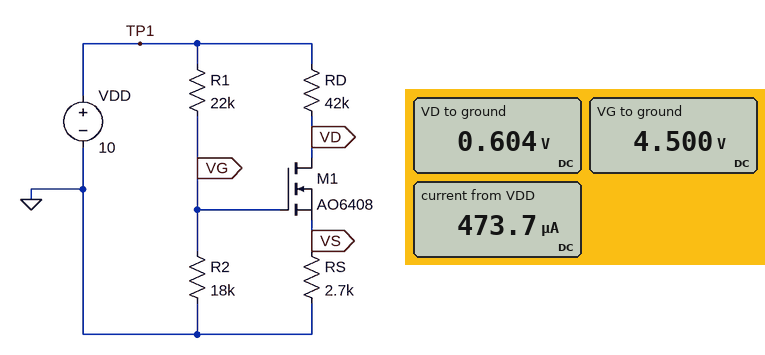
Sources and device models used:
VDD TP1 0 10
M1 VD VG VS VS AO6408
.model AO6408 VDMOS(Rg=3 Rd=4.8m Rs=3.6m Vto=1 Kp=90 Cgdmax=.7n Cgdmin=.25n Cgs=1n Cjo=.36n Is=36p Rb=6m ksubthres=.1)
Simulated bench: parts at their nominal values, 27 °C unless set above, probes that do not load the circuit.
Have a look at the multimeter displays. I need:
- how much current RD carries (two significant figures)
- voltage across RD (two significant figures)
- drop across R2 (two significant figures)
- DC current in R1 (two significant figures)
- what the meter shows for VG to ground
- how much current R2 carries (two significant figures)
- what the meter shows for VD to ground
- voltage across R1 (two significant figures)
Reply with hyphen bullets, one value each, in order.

- 220 µA
- 9.4 V
- 4.5 V
- 250 µA
- 4.500 V
- 250 µA
- 0.604 V
- 5.5 V
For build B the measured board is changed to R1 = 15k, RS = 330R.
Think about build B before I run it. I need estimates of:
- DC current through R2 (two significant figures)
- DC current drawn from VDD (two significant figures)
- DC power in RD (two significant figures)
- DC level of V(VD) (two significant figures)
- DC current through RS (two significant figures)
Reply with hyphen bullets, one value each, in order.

- 300 µA
- 540 µA
- 2.3 mW
- 78 mV
- 240 µA
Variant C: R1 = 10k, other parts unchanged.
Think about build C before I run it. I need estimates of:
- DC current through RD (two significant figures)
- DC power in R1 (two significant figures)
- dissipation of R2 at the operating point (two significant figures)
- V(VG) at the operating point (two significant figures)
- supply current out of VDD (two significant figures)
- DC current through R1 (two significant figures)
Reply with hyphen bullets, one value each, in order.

- 220 µA
- 1.3 mW
- 2.3 mW
- 6.4 V
- 580 µA
- 360 µA
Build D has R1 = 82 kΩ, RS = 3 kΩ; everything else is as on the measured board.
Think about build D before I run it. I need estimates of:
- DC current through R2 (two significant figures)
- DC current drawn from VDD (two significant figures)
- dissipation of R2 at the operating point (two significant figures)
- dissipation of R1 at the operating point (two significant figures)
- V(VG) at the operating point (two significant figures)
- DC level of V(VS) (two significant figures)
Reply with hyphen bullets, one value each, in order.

- 100 µA
- 320 µA
- 180 µW
- 820 µW
- 1.8 V
- 670 mV
